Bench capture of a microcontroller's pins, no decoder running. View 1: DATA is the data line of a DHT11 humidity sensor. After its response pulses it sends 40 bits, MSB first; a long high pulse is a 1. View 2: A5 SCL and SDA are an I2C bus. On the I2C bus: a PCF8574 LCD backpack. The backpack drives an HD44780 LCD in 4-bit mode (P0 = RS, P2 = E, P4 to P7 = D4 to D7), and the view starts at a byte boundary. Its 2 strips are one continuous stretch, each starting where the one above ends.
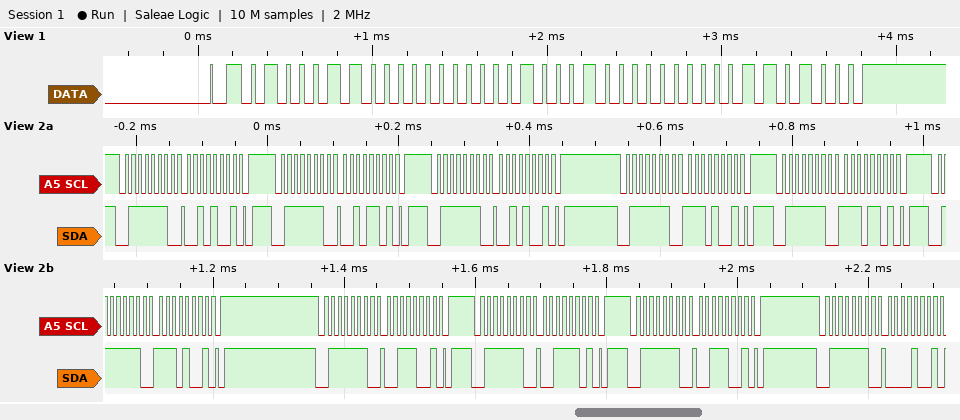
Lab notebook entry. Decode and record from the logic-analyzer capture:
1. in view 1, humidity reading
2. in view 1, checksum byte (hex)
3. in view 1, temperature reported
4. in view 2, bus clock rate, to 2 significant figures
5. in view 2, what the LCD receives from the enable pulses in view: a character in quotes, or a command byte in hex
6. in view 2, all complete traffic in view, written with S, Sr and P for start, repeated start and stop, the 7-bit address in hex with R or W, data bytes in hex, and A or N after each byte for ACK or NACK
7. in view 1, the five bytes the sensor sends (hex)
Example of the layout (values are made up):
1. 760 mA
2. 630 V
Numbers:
1. 70 %
2. 0x68
3. 34.0 °C
4. 100 kHz
5. '.'
6. S 3FW A 29 A P S 3FW A 2D A P S 3FW A 29 A P S 3FW A E9 A P S 3FW A ED A P S 3FW A E9 A P S 3FW A 39 A P S 3FW A 3D A P S 3FW A 39 A P S 3FW A 09 A
7. 46 00 22 00 68
